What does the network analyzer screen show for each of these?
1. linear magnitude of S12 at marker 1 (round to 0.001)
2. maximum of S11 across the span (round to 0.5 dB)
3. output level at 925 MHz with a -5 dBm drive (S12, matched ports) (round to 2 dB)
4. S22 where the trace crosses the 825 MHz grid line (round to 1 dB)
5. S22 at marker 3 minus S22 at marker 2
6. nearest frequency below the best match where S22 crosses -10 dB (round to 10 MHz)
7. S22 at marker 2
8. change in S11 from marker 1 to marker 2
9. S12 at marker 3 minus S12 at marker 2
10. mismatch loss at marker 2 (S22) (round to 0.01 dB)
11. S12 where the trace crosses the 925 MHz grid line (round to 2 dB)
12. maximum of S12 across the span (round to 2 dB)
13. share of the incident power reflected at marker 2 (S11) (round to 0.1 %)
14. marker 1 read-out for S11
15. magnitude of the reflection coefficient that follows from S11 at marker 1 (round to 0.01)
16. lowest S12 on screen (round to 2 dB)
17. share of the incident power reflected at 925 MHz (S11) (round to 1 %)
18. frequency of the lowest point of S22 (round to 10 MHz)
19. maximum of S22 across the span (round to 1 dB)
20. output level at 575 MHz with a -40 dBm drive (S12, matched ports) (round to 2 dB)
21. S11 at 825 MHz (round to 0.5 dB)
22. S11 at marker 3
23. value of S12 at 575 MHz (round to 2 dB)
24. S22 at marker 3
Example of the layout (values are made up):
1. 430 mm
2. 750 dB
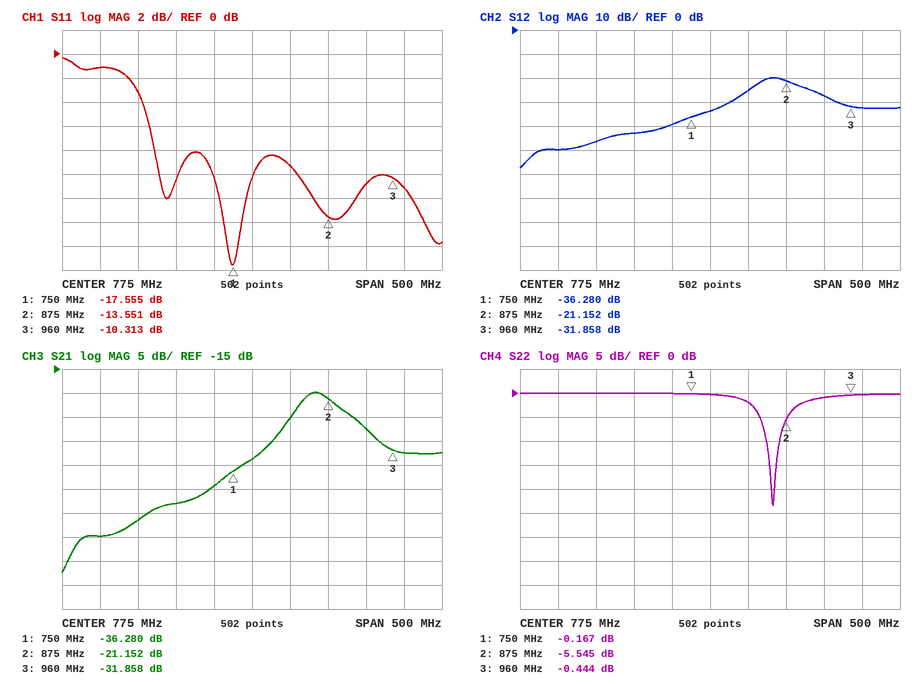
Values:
1. 0.015
2. -0.5 dB
3. -32 dBm
4. -2 dB
5. 5.101 dB
6. 850 MHz
7. -5.545 dB
8. 4.004 dB
9. -10.706 dB
10. 1.42 dB
11. -28 dB
12. -20 dB
13. 4.4 %
14. -17.555 dB
15. 0.13
16. -58 dB
17. 8 %
18. 860 MHz
19. 0 dB
20. -90 dBm
21. -9.5 dB
22. -10.313 dB
23. -50 dB
24. -0.444 dB
